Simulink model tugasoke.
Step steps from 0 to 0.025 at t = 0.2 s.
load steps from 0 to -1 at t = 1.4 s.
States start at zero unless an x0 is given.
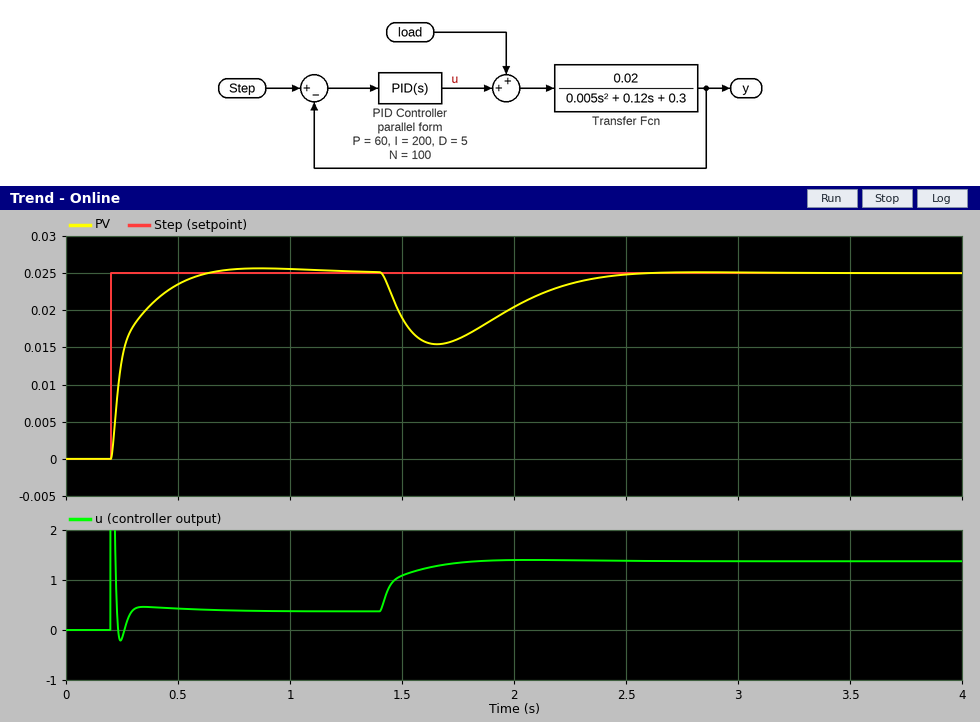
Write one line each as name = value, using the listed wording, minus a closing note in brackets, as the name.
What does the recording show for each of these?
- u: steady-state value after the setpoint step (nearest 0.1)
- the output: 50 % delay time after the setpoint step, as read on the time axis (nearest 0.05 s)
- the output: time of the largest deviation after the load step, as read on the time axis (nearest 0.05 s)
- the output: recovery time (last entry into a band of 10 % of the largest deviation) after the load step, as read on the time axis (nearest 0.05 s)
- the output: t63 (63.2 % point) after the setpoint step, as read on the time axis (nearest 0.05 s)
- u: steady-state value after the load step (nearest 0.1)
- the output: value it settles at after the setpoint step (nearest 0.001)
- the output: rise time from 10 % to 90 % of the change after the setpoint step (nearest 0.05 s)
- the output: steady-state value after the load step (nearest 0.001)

u: steady-state value after the setpoint step = 0.4
the output: 50 % delay time after the setpoint step, as read on the time axis = 0.25 s
the output: time of the largest deviation after the load step, as read on the time axis = 1.65 s
the output: recovery time (last entry into a band of 10 % of the largest deviation) after the load step, as read on the time axis = 2.30 s
the output: t63 (63.2 % point) after the setpoint step, as read on the time axis = 0.25 s
u: steady-state value after the load step = 1.4
the output: value it settles at after the setpoint step = 0.025
the output: rise time from 10 % to 90 % of the change after the setpoint step = 0.25 s
the output: steady-state value after the load step = 0.025
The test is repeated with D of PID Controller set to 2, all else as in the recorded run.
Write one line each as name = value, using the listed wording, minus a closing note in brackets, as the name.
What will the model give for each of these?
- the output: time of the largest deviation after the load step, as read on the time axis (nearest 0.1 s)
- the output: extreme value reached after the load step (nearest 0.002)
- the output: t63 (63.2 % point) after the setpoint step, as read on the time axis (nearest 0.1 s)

the output: time of the largest deviation after the load step, as read on the time axis = 1.6 s
the output: extreme value reached after the load step = 0.014
the output: t63 (63.2 % point) after the setpoint step, as read on the time axis = 0.3 s
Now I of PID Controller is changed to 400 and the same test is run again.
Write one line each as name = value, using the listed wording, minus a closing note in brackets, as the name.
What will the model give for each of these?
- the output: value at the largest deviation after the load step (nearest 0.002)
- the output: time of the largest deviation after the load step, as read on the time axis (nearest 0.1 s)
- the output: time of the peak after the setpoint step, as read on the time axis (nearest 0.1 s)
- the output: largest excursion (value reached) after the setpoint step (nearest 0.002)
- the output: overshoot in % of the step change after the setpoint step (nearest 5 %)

the output: value at the largest deviation after the load step = 0.016
the output: time of the largest deviation after the load step, as read on the time axis = 1.6 s
the output: time of the peak after the setpoint step, as read on the time axis = 0.6 s
the output: largest excursion (value reached) after the setpoint step = 0.028
the output: overshoot in % of the step change after the setpoint step = 10 %
